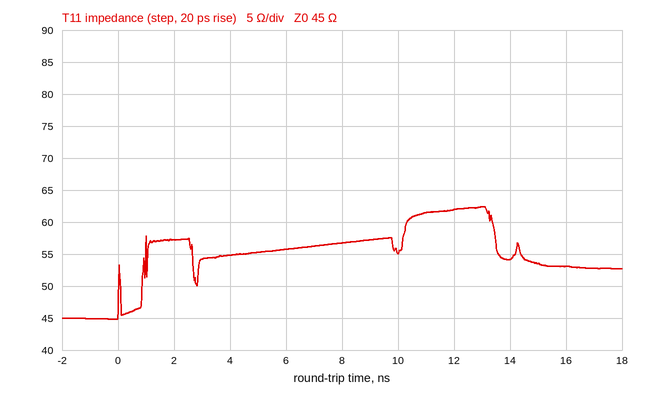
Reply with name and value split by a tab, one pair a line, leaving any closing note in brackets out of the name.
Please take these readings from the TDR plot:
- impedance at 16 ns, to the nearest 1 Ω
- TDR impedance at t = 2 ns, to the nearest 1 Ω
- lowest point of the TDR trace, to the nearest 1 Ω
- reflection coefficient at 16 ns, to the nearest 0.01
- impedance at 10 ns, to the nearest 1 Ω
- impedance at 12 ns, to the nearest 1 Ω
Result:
impedance at 16 ns, to the nearest 1 Ω	53 Ω
TDR impedance at t = 2 ns, to the nearest 1 Ω	57 Ω
lowest point of the TDR trace, to the nearest 1 Ω	45 Ω
reflection coefficient at 16 ns, to the nearest 0.01	+0.08
impedance at 10 ns, to the nearest 1 Ω	55 Ω
impedance at 12 ns, to the nearest 1 Ω	62 Ω
